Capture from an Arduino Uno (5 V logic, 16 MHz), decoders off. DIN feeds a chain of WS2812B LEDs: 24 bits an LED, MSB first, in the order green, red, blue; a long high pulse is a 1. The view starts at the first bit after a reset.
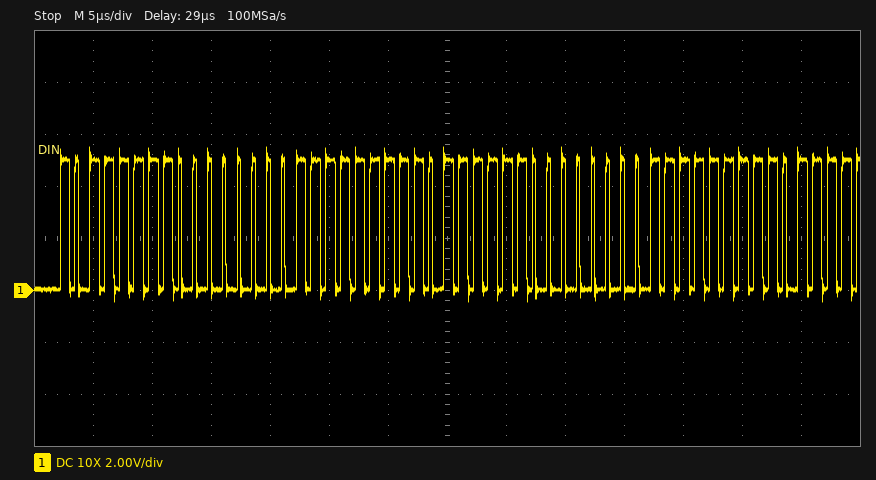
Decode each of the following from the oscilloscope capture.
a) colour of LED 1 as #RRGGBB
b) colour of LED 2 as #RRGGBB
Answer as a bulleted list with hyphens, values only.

- #00BFFF
- #00BFFF
